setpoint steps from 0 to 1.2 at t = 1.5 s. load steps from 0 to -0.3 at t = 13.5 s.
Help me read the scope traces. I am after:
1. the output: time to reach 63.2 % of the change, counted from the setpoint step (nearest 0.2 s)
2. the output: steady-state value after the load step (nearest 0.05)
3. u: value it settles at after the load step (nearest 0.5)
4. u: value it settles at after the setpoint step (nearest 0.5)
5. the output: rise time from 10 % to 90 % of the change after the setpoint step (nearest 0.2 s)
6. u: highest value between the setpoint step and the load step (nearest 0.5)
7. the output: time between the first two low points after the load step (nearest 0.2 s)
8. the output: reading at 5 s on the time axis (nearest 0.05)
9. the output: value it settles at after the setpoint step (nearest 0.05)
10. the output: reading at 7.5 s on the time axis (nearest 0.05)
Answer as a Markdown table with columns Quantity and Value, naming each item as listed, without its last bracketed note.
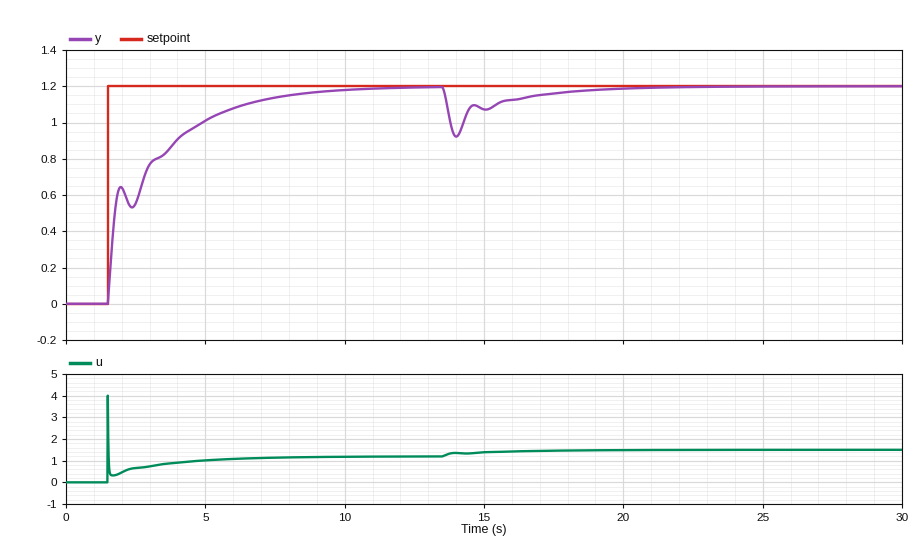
| Quantity | Value |
|---|---|
| the output: time to reach 63.2 % of the change, counted from the setpoint step | 1.4 s |
| the output: steady-state value after the load step | 1.20 |
| u: value it settles at after the load step | 1.5 |
| u: value it settles at after the setpoint step | 1.0 |
| the output: rise time from 10 % to 90 % of the change after the setpoint step | 4.4 s |
| u: highest value between the setpoint step and the load step | 4.0 |
| the output: time between the first two low points after the load step | 1.0 s |
| the output: reading at 5 s on the time axis | 1.00 |
| the output: value it settles at after the setpoint step | 1.20 |
| the output: reading at 7.5 s on the time axis | 1.15 |
